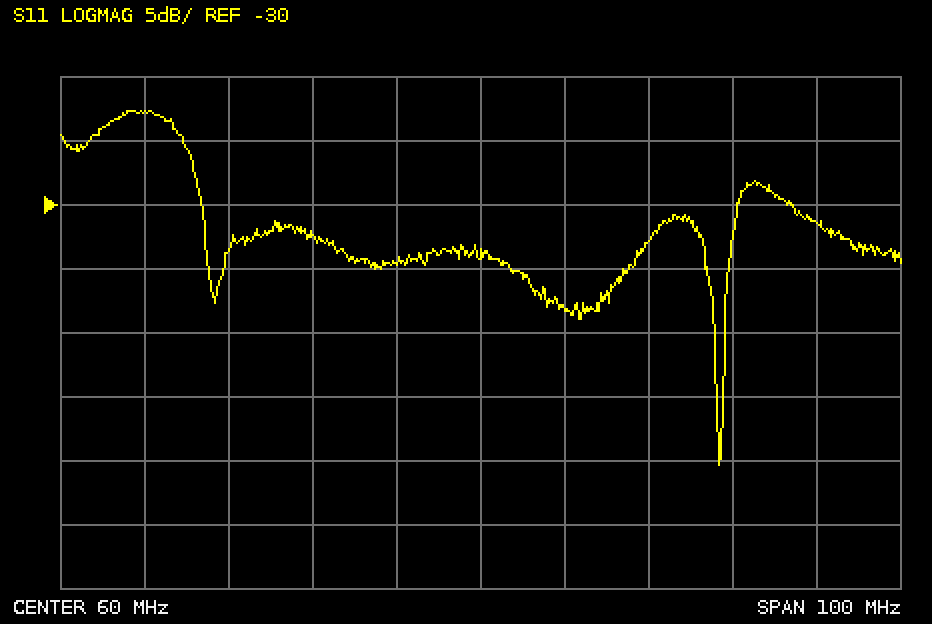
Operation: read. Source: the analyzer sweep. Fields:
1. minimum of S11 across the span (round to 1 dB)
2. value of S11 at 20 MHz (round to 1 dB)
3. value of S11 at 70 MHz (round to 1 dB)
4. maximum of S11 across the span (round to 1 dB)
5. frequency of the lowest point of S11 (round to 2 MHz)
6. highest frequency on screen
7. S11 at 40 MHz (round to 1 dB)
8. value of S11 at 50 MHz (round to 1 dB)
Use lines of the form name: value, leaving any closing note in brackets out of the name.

minimum of S11 across the span: -50 dB
value of S11 at 20 MHz: -23 dB
value of S11 at 70 MHz: -38 dB
maximum of S11 across the span: -23 dB
frequency of the lowest point of S11: 88 MHz
highest frequency on screen: 110 MHz
S11 at 40 MHz: -32 dB
value of S11 at 50 MHz: -35 dB
